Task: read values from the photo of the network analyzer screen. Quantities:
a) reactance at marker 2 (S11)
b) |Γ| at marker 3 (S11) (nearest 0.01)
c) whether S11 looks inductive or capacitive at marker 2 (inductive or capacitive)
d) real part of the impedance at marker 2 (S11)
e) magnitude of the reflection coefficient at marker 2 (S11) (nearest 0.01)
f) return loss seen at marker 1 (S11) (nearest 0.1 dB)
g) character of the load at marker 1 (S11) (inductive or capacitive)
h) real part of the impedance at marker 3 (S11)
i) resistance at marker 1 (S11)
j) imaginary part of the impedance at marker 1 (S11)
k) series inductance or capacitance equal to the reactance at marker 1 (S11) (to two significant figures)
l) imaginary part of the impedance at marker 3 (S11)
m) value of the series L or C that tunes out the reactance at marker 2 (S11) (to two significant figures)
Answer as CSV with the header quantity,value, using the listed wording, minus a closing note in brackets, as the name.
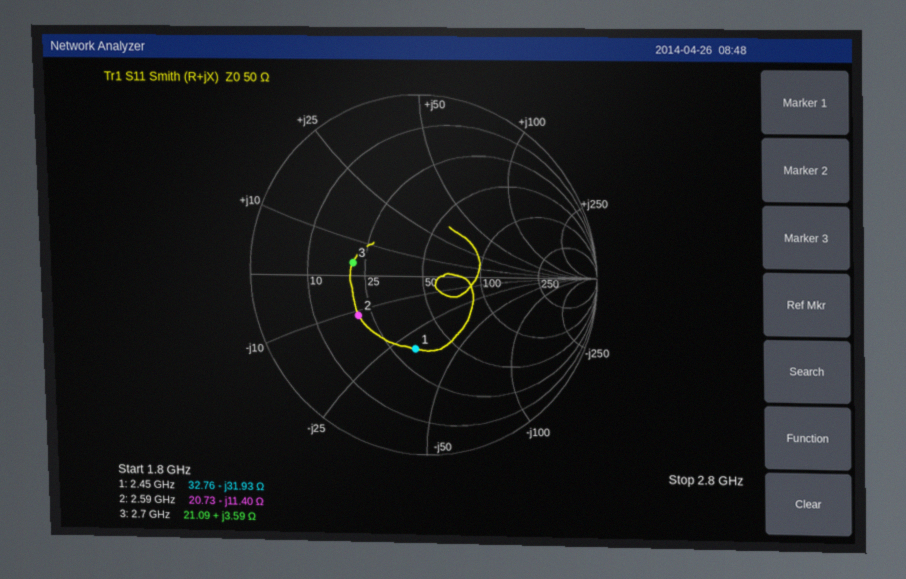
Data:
quantity,value
reactance at marker 2,-11.40 Ω
|Γ| at marker 3 (S11),0.41
whether S11 looks inductive or capacitive at marker 2,capacitive
real part of the impedance at marker 2,20.73 Ω
magnitude of the reflection coefficient at marker 2 (S11),0.44
return loss seen at marker 1 (S11),7.8 dB
character of the load at marker 1 (S11),capacitive
real part of the impedance at marker 3,21.09 Ω
resistance at marker 1,32.76 Ω
imaginary part of the impedance at marker 1,-31.93 Ω
series inductance or capacitance equal to the reactance at marker 1 (S11),2.0 pF
imaginary part of the impedance at marker 3,+3.59 Ω
value of the series L or C that tunes out the reactance at marker 2 (S11),700 pH
